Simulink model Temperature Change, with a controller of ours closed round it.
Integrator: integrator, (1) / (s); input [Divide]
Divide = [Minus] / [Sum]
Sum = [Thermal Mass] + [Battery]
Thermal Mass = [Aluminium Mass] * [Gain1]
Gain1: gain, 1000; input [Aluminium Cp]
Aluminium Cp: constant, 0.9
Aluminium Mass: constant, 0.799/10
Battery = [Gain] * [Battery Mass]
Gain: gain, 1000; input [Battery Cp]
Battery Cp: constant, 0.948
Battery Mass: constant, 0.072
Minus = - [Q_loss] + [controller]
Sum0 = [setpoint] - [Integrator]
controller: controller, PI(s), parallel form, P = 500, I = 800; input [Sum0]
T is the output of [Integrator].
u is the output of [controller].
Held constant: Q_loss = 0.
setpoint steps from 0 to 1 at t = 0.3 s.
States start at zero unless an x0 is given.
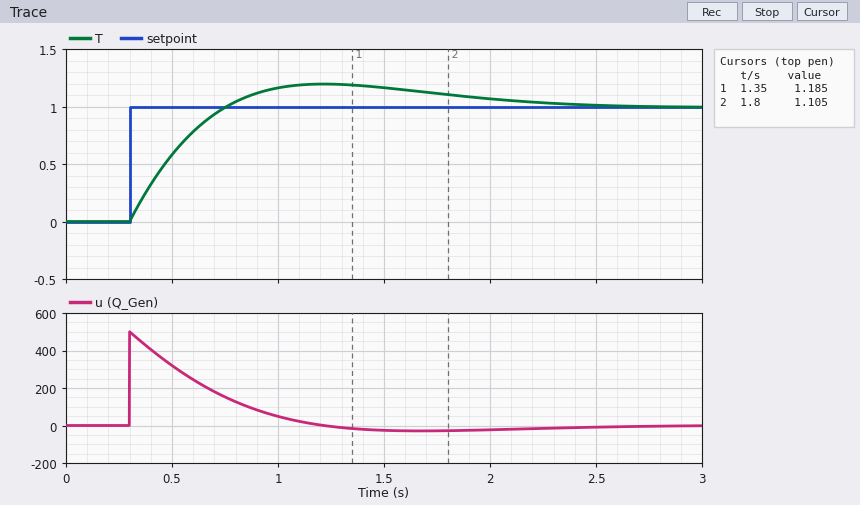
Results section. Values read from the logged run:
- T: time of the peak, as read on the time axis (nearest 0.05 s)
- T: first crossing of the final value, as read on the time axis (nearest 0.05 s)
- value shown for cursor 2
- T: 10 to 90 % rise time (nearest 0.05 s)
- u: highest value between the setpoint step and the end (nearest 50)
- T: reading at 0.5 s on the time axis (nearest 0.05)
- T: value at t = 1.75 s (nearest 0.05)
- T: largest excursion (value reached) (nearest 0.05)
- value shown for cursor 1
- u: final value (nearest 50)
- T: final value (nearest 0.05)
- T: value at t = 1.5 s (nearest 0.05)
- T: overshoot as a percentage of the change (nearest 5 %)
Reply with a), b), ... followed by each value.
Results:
a) 1.20 s
b) 0.75 s
c) 1.105
d) 0.35 s
e) 500
f) 0.60
g) 1.10
h) 1.20
i) 1.185
j) 0
k) 1.00
l) 1.15
m) 20 %
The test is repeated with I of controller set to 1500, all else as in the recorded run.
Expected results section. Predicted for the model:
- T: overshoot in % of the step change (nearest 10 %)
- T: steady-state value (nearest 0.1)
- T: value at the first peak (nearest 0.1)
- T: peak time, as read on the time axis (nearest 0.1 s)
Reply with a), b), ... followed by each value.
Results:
a) 30 %
b) 1.0
c) 1.3
d) 1.0 s
